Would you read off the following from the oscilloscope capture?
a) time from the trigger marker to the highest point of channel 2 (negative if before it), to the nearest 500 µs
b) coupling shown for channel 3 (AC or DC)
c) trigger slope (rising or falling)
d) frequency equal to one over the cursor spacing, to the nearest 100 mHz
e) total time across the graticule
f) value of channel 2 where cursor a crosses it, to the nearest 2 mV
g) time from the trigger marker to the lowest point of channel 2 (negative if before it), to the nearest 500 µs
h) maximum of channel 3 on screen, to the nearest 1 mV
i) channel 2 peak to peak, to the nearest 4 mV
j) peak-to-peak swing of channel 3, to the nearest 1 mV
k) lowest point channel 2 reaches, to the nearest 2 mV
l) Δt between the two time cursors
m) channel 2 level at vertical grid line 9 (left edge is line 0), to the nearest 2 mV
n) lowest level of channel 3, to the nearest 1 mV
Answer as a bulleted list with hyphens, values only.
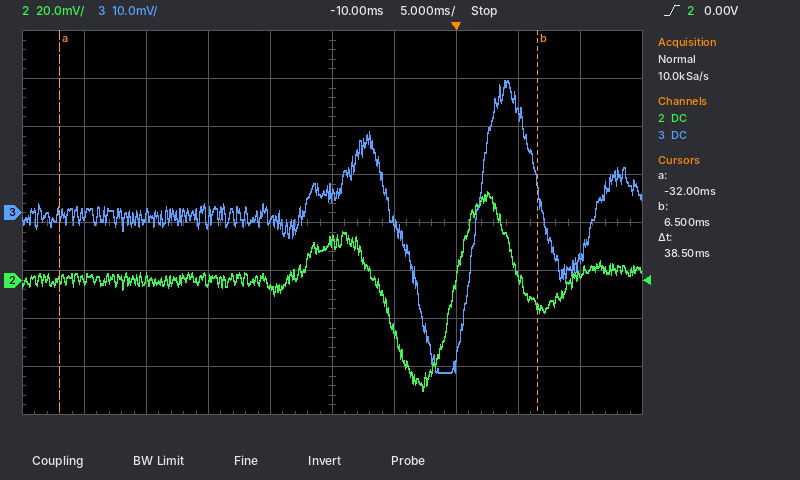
- +2.5 ms
- DC
- rising
- 26.0 Hz
- 50 ms
- 0 mV
- -2.5 ms
- 28 mV
- 84 mV
- 61 mV
- -46 mV
- 38.5 ms
- 2 mV
- -33 mV
